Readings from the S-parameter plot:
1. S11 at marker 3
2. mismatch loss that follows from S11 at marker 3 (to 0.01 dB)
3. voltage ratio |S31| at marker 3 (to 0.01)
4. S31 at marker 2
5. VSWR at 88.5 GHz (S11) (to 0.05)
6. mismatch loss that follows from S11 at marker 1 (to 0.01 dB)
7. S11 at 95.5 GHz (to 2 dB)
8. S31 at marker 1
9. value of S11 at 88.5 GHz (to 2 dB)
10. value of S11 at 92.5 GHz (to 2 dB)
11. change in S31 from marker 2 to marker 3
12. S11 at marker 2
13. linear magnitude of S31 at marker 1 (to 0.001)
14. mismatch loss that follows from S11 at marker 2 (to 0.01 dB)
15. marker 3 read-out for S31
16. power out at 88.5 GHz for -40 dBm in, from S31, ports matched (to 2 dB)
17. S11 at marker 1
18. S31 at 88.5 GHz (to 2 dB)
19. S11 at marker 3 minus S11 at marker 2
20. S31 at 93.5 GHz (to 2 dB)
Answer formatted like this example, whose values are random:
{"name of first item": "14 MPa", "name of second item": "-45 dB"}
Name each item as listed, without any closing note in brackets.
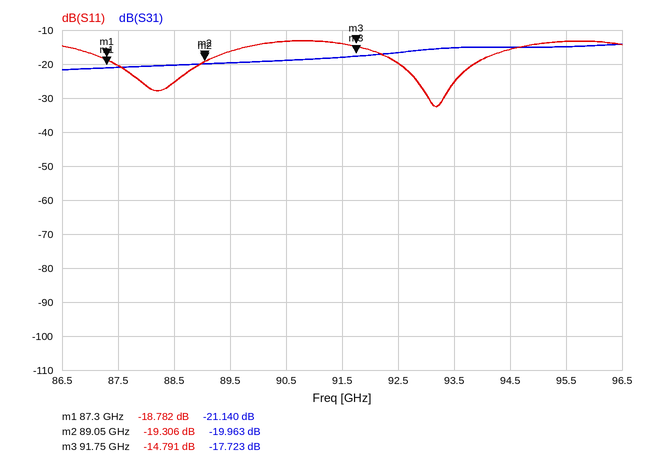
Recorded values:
{"S11 at marker 3": "-14.791 dB", "mismatch loss that follows from S11 at marker 3": "0.15 dB", "voltage ratio |S31| at marker 3": "0.13", "S31 at marker 2": "-19.963 dB", "VSWR at 88.5 GHz (S11)": "1.10", "mismatch loss that follows from S11 at marker 1": "0.06 dB", "S11 at 95.5 GHz": "-14 dB", "S31 at marker 1": "-21.140 dB", "value of S11 at 88.5 GHz": "-26 dB", "value of S11 at 92.5 GHz": "-20 dB", "change in S31 from marker 2 to marker 3": "2.240 dB", "S11 at marker 2": "-19.306 dB", "linear magnitude of S31 at marker 1": "0.088", "mismatch loss that follows from S11 at marker 2": "0.05 dB", "marker 3 read-out for S31": "-17.723 dB", "power out at 88.5 GHz for -40 dBm in, from S31, ports matched": "-60 dBm", "S11 at marker 1": "-18.782 dB", "S31 at 88.5 GHz": "-20 dB", "S11 at marker 3 minus S11 at marker 2": "4.515 dB", "S31 at 93.5 GHz": "-16 dB"}
